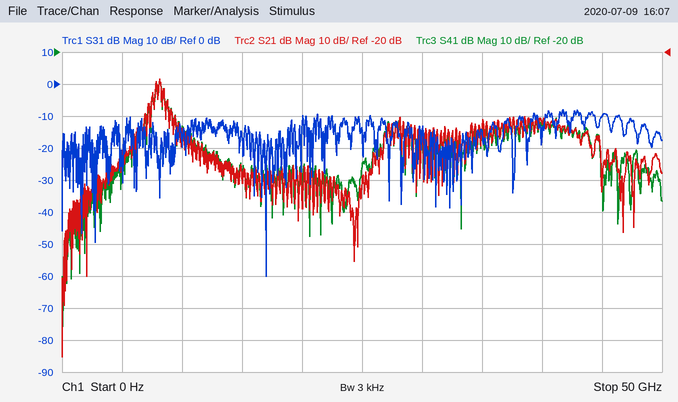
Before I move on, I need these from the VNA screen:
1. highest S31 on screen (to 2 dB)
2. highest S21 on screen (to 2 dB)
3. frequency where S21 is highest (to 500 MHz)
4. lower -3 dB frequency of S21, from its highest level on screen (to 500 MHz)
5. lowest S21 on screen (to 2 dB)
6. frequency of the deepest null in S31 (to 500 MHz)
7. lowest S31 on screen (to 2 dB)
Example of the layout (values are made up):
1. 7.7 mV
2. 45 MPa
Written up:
1. -8 dB
2. -28 dB
3. 8.0 GHz
4. 8.0 GHz
5. -116 dB
6. 17.0 GHz
7. -60 dB
